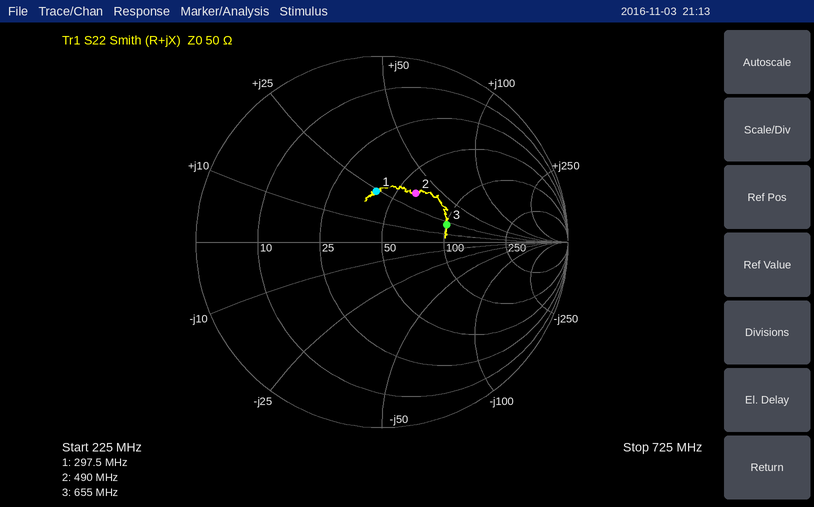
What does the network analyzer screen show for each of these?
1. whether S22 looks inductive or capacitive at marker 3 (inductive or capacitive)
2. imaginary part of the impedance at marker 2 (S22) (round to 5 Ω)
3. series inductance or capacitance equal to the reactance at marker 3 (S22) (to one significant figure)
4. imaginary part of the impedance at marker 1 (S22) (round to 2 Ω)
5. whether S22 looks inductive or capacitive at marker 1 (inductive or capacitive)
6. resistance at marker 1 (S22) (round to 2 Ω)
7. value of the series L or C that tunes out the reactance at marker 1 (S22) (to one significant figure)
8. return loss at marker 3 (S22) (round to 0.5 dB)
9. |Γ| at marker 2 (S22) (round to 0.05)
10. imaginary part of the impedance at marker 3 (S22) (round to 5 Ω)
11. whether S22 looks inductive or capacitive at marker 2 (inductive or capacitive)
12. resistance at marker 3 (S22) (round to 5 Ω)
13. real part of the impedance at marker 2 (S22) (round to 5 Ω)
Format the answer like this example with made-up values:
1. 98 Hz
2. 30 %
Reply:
1. inductive
2. +35 Ω
3. 5 nH
4. +24 Ω
5. inductive
6. 40 Ω
7. 20 pF
8. 9.0 dB
9. 0.30
10. +20 Ω
11. inductive
12. 100 Ω
13. 60 Ω
